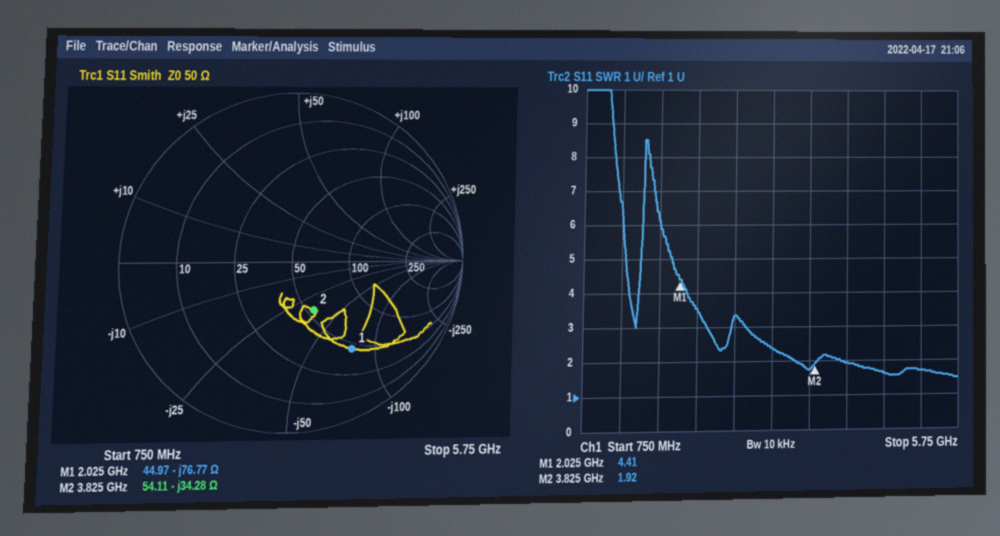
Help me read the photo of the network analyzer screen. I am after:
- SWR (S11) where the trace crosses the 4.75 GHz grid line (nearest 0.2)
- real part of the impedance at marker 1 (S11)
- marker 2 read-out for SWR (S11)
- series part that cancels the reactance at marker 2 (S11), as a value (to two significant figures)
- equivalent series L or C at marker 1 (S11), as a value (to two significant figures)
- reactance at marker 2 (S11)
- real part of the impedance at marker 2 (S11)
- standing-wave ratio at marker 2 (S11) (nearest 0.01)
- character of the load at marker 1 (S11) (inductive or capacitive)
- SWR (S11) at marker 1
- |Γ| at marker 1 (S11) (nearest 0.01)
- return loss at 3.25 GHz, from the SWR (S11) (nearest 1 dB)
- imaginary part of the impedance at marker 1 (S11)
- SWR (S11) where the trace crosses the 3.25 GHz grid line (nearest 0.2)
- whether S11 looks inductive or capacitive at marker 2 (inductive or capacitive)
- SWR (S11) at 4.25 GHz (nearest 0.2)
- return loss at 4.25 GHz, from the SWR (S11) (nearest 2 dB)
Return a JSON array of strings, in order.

["1.6", "44.97 Ω", "1.92", "1.4 nH", "1.0 pF", "-34.28 Ω", "54.11 Ω", "1.92", "capacitive", "4.41", "0.63", "8 dB", "-76.77 Ω", "2.4", "capacitive", "2.0", "10 dB"]
